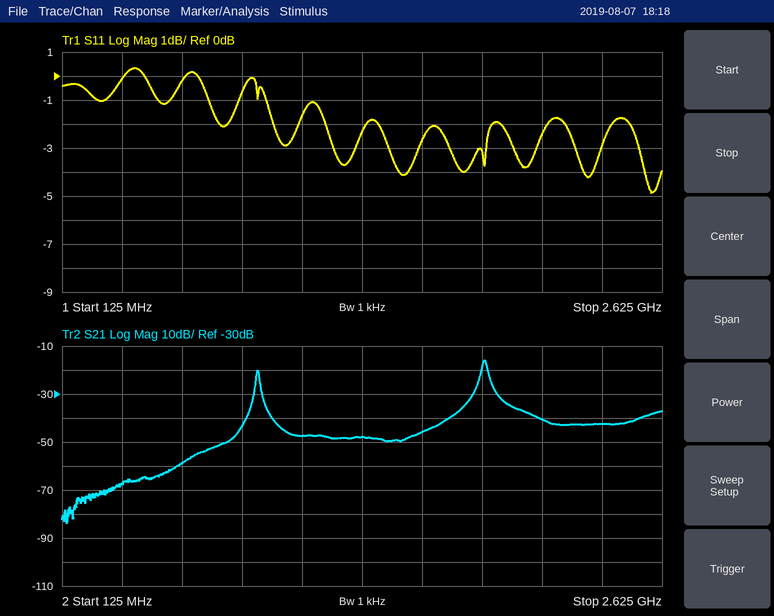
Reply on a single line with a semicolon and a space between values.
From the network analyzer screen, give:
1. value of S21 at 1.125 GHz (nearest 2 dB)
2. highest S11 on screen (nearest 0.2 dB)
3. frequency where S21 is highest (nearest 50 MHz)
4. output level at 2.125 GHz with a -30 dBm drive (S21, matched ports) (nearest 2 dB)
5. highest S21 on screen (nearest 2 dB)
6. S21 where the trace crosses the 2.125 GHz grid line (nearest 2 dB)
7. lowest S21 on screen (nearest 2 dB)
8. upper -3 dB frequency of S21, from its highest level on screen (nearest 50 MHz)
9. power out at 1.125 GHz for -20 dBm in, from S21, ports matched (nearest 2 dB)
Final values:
-48 dB; 0.4 dB; 1.90 GHz; -70 dBm; -16 dB; -40 dB; -84 dB; 1.90 GHz; -68 dBm
